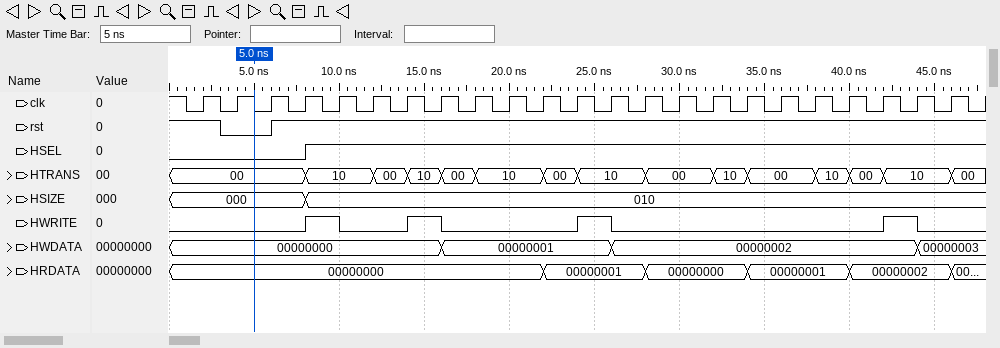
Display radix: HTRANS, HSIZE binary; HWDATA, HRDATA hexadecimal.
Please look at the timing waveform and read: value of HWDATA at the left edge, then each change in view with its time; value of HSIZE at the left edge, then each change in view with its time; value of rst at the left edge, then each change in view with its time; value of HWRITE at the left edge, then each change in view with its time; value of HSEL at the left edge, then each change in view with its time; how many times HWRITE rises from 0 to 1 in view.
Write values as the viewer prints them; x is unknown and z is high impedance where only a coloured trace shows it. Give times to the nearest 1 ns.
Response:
00000000, 00000001 at 16 ns, 00000002 at 26 ns, 00000003 at 44 ns
000, 010 at 8 ns
1, 0 at 3 ns, 1 at 6 ns
0, 1 at 8 ns, 0 at 10 ns, 1 at 14 ns, 0 at 16 ns, 1 at 24 ns, 0 at 26 ns, 1 at 42 ns, 0 at 44 ns
0, 1 at 8 ns
4
